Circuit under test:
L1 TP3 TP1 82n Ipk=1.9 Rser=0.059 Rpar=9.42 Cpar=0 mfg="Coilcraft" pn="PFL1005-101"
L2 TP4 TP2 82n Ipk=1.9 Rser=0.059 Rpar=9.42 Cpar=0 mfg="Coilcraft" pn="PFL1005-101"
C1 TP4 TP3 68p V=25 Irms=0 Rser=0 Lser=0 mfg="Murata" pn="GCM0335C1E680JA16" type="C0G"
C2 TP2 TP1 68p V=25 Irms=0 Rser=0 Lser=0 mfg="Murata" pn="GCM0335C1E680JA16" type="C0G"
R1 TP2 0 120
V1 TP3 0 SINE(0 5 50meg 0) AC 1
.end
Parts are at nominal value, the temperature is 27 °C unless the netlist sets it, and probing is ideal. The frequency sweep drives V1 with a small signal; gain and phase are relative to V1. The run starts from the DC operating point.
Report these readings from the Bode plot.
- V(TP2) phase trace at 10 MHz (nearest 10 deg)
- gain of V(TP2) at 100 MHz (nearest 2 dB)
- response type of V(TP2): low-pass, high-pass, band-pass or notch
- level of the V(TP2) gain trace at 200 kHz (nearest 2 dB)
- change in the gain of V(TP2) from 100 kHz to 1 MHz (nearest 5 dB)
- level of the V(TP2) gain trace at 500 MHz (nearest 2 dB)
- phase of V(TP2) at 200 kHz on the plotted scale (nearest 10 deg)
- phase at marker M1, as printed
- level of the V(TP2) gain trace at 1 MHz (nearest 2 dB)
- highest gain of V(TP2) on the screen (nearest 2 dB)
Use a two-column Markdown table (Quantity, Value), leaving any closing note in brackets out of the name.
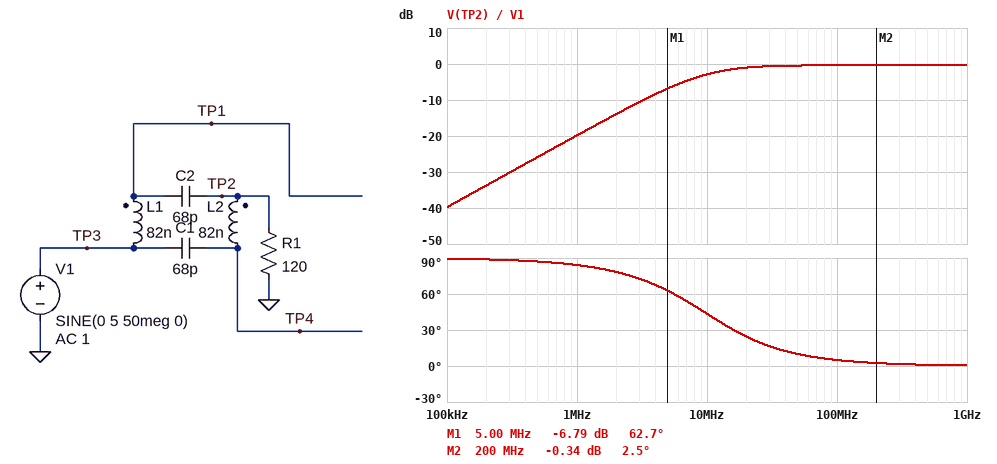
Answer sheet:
| Quantity | Value |
|---|---|
| V(TP2) phase trace at 10 MHz | 40 deg |
| gain of V(TP2) at 100 MHz | 0 dB |
| response type of V(TP2): low-pass, high-pass, band-pass or notch | high-pass |
| level of the V(TP2) gain trace at 200 kHz | -34 dB |
| change in the gain of V(TP2) from 100 kHz to 1 MHz | 20 dB |
| level of the V(TP2) gain trace at 500 MHz | 0 dB |
| phase of V(TP2) at 200 kHz on the plotted scale | 90 deg |
| phase at marker M1, as printed | 62.7 deg |
| level of the V(TP2) gain trace at 1 MHz | -20 dB |
| highest gain of V(TP2) on the screen | 0 dB |
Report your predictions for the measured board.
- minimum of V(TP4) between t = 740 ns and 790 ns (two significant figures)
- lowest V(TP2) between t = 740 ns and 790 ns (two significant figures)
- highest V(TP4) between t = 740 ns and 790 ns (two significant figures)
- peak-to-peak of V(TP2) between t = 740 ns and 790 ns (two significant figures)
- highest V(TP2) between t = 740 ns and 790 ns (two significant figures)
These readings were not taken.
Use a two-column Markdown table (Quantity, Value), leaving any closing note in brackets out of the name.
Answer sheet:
| Quantity | Value |
|---|---|
| minimum of V(TP4) between t = 740 ns and 790 ns | -4.9 V |
| lowest V(TP2) between t = 740 ns and 790 ns | -4.8 V |
| highest V(TP4) between t = 740 ns and 790 ns | 4.9 V |
| peak-to-peak of V(TP2) between t = 740 ns and 790 ns | 9.5 V |
| highest V(TP2) between t = 740 ns and 790 ns | 4.8 V |
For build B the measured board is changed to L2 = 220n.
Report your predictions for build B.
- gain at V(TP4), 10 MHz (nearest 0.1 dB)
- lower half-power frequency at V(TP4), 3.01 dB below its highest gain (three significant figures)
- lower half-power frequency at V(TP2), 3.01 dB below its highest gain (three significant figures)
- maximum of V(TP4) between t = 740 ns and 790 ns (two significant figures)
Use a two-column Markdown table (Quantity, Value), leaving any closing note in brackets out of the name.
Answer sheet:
| Quantity | Value |
|---|---|
| gain at V(TP4), 10 MHz | -2.7 dB |
| lower half-power frequency at V(TP4), 3.01 dB below its highest gain | 9.27 MHz |
| lower half-power frequency at V(TP2), 3.01 dB below its highest gain | 9.04 MHz |
| maximum of V(TP4) between t = 740 ns and 790 ns | 4.9 V |
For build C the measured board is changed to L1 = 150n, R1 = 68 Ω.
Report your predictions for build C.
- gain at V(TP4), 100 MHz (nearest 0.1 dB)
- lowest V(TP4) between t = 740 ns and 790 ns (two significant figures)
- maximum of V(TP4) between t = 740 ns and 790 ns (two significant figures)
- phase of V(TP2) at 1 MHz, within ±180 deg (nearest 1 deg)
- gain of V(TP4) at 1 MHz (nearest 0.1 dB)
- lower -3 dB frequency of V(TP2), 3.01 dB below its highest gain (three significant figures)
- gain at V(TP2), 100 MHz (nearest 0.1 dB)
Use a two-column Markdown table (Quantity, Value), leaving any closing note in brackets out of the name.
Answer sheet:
| Quantity | Value |
|---|---|
| gain at V(TP4), 100 MHz | -0.1 dB |
| lowest V(TP4) between t = 740 ns and 790 ns | -4.8 V |
| maximum of V(TP4) between t = 740 ns and 790 ns | 4.8 V |
| phase of V(TP2) at 1 MHz, within ±180 deg | 87 deg |
| gain of V(TP4) at 1 MHz | -24.7 dB |
| lower -3 dB frequency of V(TP2), 3.01 dB below its highest gain | 15.2 MHz |
| gain at V(TP2), 100 MHz | -0.7 dB |
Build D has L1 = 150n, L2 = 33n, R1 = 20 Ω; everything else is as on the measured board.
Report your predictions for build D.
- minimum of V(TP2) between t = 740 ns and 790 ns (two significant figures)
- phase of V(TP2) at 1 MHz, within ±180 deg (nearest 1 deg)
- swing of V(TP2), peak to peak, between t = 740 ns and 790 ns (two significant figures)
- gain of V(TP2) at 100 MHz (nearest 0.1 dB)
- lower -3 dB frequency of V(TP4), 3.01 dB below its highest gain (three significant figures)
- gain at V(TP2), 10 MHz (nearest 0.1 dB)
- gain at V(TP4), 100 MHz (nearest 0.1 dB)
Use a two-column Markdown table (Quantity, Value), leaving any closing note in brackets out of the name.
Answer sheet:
| Quantity | Value |
|---|---|
| minimum of V(TP2) between t = 740 ns and 790 ns | -3.1 V |
| phase of V(TP2) at 1 MHz, within ±180 deg | 89 deg |
| swing of V(TP2), peak to peak, between t = 740 ns and 790 ns | 6.2 V |
| gain of V(TP2) at 100 MHz | -2.4 dB |
| lower -3 dB frequency of V(TP4), 3.01 dB below its highest gain | 49.7 MHz |
| gain at V(TP2), 10 MHz | -15.4 dB |
| gain at V(TP4), 100 MHz | -0.8 dB |
